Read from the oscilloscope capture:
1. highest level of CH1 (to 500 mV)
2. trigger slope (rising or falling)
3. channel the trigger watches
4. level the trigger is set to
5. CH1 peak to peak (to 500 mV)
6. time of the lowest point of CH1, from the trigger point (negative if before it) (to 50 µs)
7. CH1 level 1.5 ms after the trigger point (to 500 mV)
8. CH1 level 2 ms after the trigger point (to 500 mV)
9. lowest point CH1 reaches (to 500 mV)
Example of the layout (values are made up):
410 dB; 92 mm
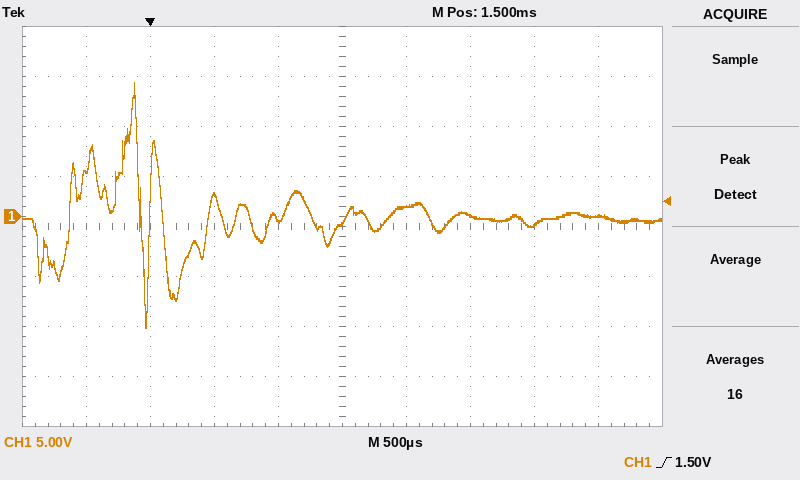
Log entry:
13.5 V; rising; CH1; 1.50 V; 24.5 V; -50 µs; -500 mV; 1.0 V; -11.0 V
